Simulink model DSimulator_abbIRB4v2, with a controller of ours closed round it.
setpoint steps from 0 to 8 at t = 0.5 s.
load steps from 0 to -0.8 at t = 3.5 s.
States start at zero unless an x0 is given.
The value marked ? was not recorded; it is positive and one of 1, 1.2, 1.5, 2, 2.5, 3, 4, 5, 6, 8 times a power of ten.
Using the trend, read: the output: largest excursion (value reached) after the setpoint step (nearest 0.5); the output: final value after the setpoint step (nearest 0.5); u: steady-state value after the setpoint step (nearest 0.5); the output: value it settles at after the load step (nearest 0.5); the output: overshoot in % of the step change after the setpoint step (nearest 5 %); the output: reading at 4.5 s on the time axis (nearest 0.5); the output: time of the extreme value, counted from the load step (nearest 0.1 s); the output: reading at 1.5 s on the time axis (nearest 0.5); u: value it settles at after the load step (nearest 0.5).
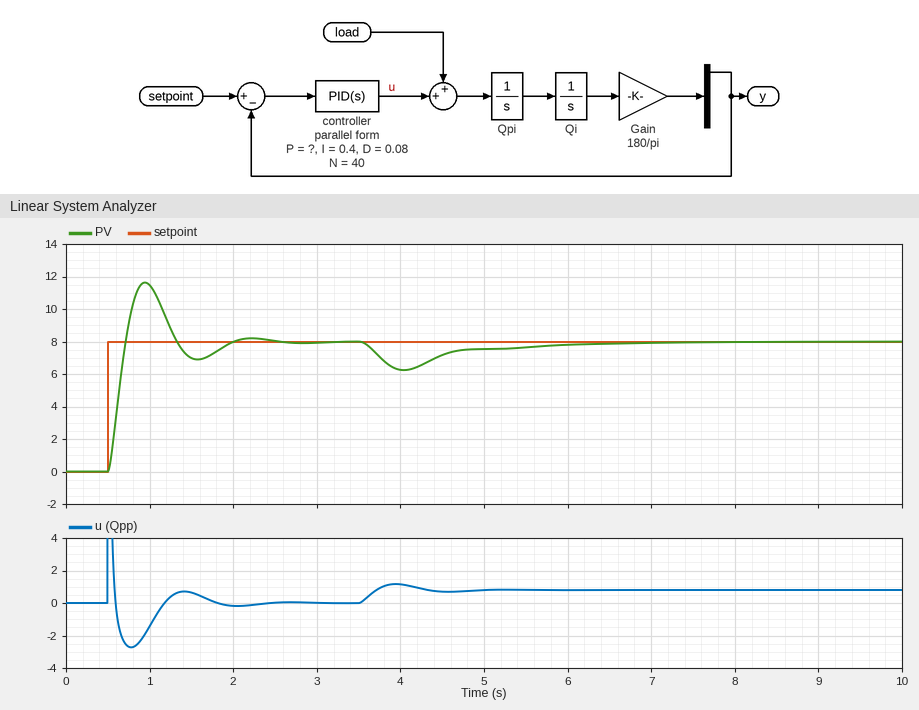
11.5
8.0
0.0
8.0
45 %
7.0
0.5 s
7.0
1.0
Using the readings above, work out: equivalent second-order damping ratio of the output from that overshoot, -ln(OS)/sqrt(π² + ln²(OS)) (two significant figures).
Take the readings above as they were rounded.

0.25
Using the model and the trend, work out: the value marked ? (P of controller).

0.5
